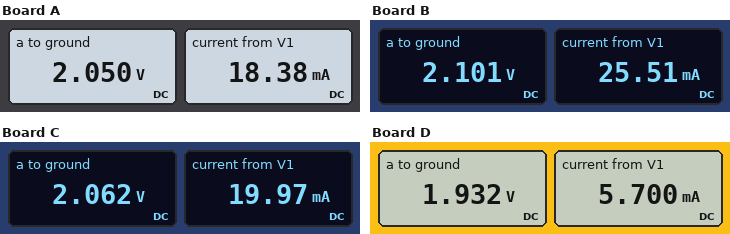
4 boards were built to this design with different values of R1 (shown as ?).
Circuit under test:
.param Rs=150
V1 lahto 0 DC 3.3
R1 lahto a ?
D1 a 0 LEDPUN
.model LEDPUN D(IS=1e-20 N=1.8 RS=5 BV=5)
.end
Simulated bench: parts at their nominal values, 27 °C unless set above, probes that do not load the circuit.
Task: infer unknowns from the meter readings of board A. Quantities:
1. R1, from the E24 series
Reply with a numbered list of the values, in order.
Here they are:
1. 68 Ω
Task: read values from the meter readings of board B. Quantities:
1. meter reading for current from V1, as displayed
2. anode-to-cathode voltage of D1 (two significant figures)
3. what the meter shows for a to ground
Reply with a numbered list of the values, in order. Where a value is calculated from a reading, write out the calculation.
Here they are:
1. 25.51 mA
2. 2.101 V = 2.1 V
3. 2.101 V
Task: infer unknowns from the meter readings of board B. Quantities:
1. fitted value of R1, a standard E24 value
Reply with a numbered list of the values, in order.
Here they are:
1. 47 Ω
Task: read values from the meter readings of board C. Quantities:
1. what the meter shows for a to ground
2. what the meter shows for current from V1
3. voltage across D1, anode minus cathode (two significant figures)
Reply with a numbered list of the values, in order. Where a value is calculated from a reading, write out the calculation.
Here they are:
1. 2.062 V
2. 19.97 mA
3. 2.062 V = 2.1 V
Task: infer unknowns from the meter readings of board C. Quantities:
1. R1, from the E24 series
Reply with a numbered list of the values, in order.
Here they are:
1. 62 Ω
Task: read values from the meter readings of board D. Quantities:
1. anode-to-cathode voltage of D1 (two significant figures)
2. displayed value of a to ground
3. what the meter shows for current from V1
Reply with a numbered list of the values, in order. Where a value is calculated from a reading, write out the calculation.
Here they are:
1. 1.932 V = 1.9 V
2. 1.932 V
3. 5.700 mA
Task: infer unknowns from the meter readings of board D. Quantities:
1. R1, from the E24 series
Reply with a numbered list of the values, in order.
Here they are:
1. 240 Ω
